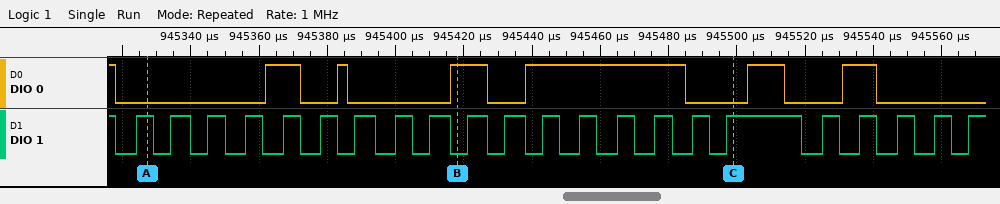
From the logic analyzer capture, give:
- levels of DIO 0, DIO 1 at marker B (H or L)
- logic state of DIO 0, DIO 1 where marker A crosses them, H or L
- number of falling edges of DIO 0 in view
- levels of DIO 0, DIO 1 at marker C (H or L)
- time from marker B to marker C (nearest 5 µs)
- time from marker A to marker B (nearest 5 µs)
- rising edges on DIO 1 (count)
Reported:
DIO 0=H, DIO 1=L
DIO 0=L, DIO 1=H
7
DIO 0=L, DIO 1=H
80 µs
90 µs
22
